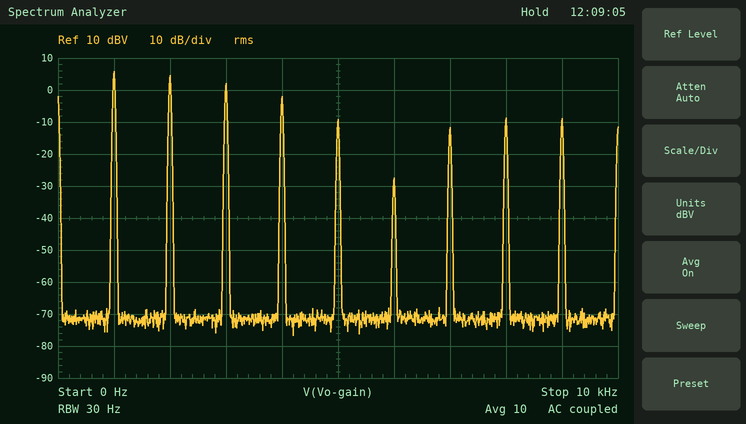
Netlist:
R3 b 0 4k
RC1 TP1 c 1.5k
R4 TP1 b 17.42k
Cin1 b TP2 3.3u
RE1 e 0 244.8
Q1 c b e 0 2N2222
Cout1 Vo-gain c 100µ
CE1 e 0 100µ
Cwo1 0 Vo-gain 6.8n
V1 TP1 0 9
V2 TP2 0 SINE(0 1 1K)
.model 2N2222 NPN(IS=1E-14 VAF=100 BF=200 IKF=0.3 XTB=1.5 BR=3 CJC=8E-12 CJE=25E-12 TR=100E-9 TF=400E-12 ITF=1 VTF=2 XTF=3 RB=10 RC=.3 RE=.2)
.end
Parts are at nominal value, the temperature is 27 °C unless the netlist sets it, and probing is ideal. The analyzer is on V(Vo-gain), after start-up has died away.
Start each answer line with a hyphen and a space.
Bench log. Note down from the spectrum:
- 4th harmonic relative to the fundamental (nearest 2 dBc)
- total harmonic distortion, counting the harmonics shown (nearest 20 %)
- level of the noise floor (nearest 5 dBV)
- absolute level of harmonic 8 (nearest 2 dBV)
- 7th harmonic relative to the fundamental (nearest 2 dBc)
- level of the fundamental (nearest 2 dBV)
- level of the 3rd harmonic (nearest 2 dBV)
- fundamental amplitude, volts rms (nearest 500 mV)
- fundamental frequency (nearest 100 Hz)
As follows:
- -8 dBc
- 120 %
- -70 dBV
- -8 dBV
- -18 dBc
- 6 dBV
- 2 dBV
- 2.0 V
- 1.0 kHz
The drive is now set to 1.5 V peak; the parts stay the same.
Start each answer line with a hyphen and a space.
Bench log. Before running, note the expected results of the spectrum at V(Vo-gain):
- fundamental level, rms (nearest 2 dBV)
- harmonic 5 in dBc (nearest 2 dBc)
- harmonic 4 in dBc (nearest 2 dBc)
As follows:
- 6 dBV
- -12 dBc
- -6 dBc
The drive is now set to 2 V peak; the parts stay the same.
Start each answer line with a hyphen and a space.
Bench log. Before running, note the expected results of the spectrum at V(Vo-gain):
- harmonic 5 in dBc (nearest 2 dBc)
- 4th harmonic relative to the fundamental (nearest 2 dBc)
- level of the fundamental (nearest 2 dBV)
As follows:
- -10 dBc
- -6 dBc
- 4 dBV
